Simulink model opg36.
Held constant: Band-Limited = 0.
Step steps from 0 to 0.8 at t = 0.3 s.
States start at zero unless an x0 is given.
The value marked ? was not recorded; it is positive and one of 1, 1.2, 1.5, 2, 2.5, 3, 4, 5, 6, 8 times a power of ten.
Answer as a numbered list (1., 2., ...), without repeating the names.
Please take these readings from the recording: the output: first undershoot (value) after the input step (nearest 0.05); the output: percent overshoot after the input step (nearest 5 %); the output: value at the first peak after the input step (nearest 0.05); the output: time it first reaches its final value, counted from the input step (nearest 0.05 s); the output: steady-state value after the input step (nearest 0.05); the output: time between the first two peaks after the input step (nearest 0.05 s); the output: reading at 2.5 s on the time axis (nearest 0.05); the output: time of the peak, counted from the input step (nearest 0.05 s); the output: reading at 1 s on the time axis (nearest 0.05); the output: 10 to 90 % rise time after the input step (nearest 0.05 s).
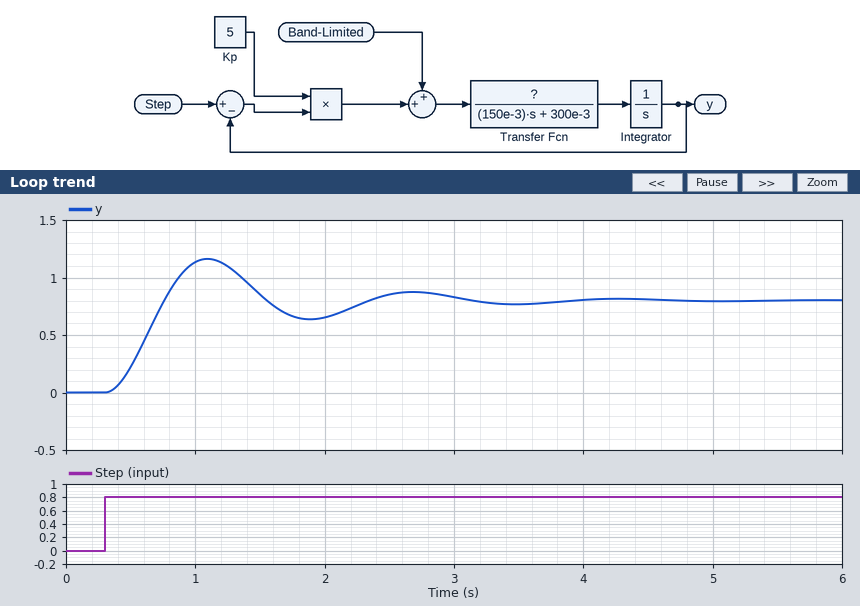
1. 0.65
2. 45 %
3. 1.15
4. 0.45 s
5. 0.80
6. 1.60 s
7. 0.85
8. 0.80 s
9. 1.15
10. 0.30 s
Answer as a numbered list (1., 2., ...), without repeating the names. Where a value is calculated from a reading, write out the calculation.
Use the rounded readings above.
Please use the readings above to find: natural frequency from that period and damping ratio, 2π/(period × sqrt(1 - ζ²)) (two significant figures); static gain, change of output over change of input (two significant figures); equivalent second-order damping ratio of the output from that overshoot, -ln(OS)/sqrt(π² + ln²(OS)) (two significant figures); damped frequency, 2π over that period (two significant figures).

1. 2π / (1.6 × sqrt(1 - 0.25²)) = 4.1 rad/s
2. (0.8 - 0) / (0.8 - 0) = 1.0
3. ln(0.45) = -0.799; 0.799 / sqrt(9.870 + 0.638) = 0.25
4. 2π / 1.6 = 3.9 rad/s
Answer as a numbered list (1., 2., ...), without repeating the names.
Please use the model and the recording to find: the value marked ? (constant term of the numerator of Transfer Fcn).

1. 0.5
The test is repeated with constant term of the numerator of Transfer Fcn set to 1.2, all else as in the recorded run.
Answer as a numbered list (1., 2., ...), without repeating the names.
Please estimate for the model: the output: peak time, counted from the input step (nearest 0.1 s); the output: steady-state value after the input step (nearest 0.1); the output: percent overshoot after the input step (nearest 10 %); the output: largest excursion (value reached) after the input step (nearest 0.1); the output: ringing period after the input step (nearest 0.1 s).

1. 0.5 s
2. 0.8
3. 60 %
4. 1.3
5. 1.0 s
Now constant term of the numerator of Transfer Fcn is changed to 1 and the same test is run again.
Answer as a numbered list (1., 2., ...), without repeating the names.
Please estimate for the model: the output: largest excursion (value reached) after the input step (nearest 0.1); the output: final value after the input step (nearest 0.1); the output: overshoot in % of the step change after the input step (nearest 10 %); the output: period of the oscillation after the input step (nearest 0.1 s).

1. 1.3
2. 0.8
3. 60 %
4. 1.1 s
